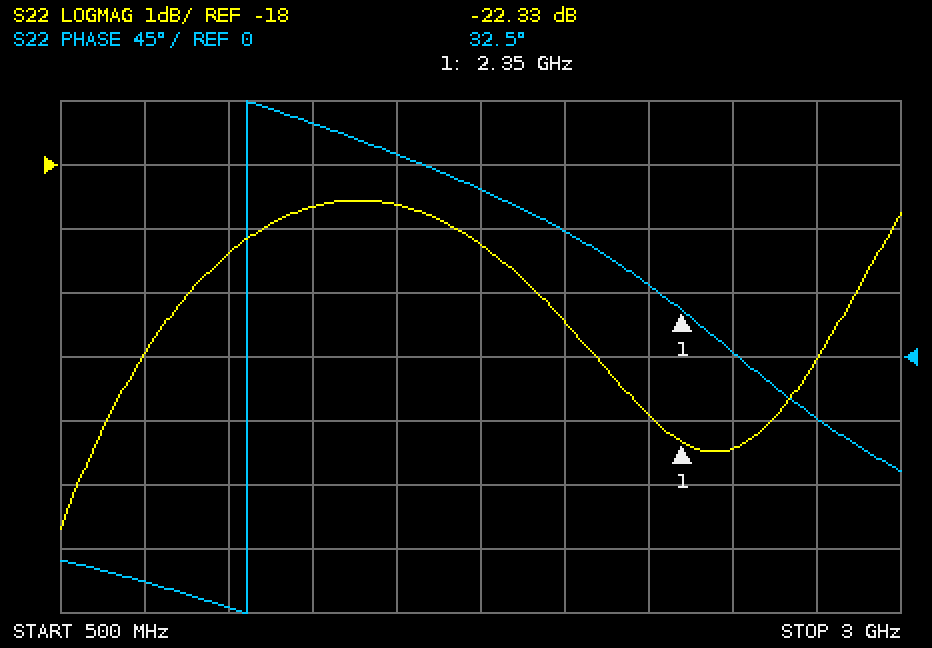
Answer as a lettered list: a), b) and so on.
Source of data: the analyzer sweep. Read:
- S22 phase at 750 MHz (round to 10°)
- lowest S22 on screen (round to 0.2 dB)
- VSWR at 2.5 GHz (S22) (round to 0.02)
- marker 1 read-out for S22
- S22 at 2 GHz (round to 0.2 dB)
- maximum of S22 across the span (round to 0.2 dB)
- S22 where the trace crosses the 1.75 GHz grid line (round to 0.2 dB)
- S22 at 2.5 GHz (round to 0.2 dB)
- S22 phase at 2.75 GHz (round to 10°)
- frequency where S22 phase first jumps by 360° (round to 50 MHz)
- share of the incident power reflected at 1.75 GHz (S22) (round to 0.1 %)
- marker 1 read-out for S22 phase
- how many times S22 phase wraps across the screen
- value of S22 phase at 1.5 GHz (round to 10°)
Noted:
a) -160°
b) -23.6 dB
c) 1.16
d) -22.33 dB
e) -20.4 dB
f) -18.6 dB
g) -19.2 dB
h) -22.4 dB
i) -40°
j) 1.05 GHz
k) 1.2 %
l) 32.5°
m) 1
n) 140°
